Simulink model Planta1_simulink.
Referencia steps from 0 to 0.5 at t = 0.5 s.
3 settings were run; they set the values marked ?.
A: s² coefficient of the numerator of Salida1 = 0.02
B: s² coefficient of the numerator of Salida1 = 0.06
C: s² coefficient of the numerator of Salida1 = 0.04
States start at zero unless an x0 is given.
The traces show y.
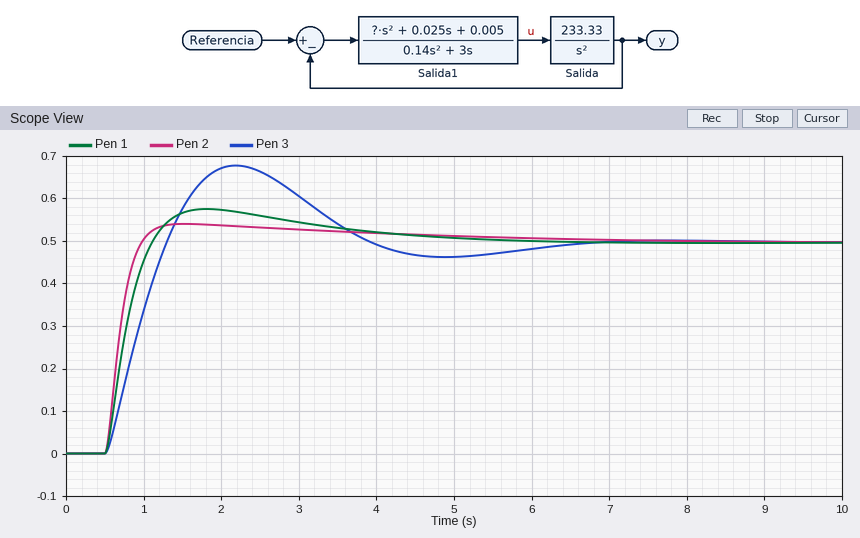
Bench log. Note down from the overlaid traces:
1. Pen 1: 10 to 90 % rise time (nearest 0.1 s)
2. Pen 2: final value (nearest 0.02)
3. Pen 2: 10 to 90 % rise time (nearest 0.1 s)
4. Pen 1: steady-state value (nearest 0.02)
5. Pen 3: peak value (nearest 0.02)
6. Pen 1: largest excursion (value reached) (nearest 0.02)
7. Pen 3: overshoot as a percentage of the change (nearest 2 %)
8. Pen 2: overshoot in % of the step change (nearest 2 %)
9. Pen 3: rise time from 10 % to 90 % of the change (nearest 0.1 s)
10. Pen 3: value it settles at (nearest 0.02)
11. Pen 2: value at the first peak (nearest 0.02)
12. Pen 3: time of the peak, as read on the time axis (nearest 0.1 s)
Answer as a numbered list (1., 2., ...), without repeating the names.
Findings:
1. 0.4 s
2. 0.50
3. 0.3 s
4. 0.50
5. 0.68
6. 0.58
7. 36 %
8. 8 %
9. 0.6 s
10. 0.50
11. 0.54
12. 2.2 s
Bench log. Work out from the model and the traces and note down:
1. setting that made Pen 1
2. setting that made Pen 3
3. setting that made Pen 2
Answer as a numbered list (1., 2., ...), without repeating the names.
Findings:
1. C
2. A
3. B
